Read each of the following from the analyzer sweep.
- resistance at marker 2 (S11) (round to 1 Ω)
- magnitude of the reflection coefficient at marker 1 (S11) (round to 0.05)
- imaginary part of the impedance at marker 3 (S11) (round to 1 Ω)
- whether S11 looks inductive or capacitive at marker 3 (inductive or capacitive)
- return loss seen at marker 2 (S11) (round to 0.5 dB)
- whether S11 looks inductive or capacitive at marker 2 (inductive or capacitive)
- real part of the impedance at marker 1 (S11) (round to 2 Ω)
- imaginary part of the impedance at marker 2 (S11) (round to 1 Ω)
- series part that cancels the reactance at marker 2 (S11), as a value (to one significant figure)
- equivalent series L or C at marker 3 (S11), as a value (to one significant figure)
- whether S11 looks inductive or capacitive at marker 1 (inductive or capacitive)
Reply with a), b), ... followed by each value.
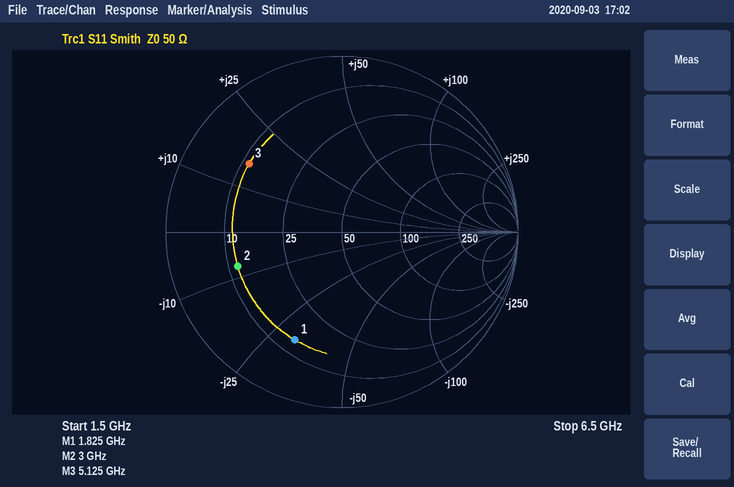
a) 12 Ω
b) 0.65
c) +16 Ω
d) inductive
e) 4.0 dB
f) capacitive
g) 14 Ω
h) -8 Ω
i) 400 pH
j) 500 pH
k) capacitive
